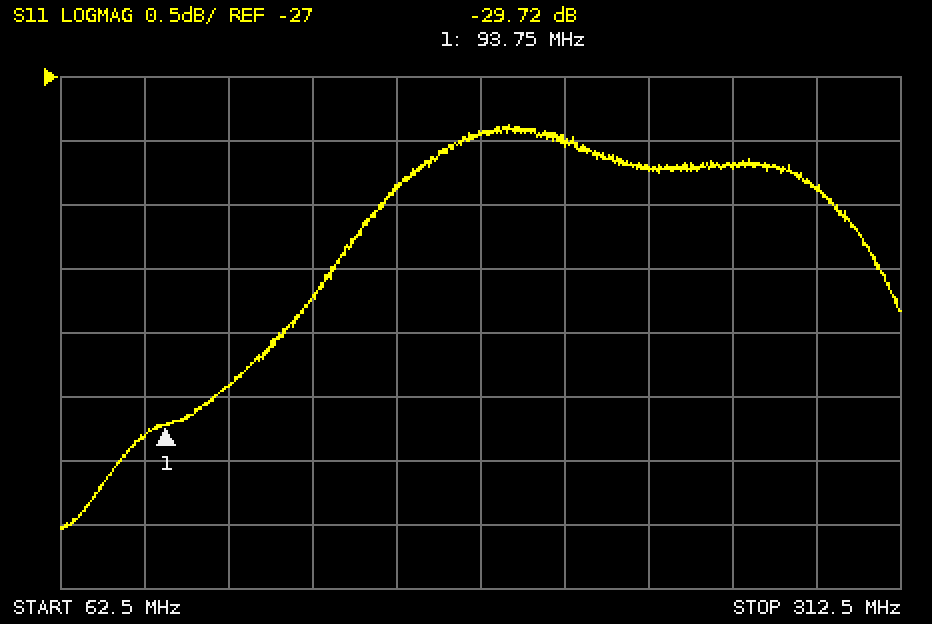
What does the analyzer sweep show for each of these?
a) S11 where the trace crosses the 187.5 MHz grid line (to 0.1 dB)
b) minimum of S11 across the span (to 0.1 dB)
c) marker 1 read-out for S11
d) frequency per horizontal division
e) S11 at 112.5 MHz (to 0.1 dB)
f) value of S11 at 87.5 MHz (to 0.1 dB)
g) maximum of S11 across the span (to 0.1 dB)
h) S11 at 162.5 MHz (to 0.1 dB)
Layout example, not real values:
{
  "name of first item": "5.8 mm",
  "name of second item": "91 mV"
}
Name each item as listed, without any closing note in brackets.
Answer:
{
  "S11 where the trace crosses the 187.5 MHz grid line": "-27.4 dB",
  "minimum of S11 across the span": "-30.5 dB",
  "marker 1 read-out for S11": "-29.72 dB",
  "frequency per horizontal division": "25 MHz",
  "S11 at 112.5 MHz": "-29.4 dB",
  "value of S11 at 87.5 MHz": "-29.8 dB",
  "maximum of S11 across the span": "-27.4 dB",
  "S11 at 162.5 MHz": "-27.9 dB"
}
